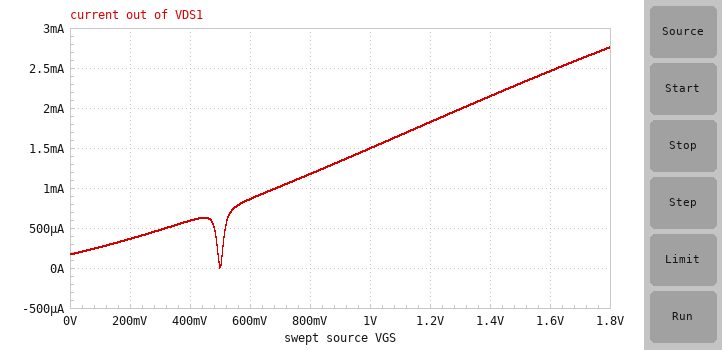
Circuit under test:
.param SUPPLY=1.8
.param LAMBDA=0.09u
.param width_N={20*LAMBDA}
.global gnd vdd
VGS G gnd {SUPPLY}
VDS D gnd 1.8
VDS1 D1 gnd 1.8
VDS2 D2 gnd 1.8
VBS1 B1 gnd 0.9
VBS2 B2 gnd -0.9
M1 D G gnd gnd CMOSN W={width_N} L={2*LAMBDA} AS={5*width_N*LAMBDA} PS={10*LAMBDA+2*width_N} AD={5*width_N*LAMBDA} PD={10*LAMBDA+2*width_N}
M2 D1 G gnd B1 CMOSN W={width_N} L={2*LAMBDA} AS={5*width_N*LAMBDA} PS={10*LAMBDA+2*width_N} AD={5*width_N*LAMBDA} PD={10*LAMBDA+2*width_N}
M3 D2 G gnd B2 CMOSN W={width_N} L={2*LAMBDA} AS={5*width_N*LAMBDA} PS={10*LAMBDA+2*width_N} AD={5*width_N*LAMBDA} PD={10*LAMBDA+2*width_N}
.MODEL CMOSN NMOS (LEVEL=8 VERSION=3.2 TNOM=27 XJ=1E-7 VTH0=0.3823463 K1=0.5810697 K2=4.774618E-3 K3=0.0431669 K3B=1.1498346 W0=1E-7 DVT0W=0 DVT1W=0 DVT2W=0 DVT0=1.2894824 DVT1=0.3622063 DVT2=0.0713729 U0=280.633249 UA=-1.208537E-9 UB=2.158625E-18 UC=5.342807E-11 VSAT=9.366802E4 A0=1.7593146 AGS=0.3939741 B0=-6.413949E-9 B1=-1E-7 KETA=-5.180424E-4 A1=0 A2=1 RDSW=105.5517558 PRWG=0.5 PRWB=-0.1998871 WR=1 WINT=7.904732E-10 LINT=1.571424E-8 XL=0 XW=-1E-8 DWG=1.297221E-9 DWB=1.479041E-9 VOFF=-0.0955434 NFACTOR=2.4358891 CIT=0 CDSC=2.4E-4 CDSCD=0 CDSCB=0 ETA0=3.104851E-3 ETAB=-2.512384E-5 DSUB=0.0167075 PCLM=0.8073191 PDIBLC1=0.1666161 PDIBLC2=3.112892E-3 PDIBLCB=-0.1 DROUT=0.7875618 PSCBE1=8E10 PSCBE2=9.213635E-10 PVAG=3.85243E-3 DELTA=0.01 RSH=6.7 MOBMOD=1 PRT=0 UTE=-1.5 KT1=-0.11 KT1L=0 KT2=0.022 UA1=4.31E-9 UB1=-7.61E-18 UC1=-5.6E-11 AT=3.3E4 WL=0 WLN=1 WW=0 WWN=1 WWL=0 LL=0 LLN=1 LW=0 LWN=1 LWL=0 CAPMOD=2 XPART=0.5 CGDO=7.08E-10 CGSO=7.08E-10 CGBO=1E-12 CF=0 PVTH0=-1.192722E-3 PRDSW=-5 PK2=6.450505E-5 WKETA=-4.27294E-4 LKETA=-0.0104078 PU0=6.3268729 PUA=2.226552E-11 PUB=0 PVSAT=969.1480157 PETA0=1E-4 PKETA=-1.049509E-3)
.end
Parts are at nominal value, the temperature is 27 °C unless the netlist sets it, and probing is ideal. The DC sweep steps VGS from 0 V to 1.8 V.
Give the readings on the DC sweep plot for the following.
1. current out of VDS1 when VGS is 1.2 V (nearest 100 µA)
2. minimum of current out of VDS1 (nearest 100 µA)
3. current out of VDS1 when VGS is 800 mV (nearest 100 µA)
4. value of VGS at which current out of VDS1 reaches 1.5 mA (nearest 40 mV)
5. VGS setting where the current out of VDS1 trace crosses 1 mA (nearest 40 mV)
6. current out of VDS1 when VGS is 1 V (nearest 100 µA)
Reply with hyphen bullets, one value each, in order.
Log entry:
- 1.8 mA
- 0 A
- 1.2 mA
- 1.00 V
- 680 mV
- 1.5 mA
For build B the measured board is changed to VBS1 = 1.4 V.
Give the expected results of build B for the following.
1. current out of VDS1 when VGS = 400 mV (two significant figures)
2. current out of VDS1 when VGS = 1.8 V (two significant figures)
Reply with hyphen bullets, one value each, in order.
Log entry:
- 580 µA
- 2.7 mA
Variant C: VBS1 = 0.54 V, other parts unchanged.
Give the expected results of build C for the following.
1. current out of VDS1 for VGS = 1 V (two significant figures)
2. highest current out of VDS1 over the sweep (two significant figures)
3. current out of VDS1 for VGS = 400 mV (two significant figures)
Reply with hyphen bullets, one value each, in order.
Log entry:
- 1.6 mA
- 2.8 mA
- 610 µA
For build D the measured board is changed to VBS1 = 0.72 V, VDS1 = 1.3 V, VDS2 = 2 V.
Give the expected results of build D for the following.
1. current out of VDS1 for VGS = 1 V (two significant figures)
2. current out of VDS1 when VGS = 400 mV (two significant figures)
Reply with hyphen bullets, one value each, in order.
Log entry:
- 1.2 mA
- 420 µA
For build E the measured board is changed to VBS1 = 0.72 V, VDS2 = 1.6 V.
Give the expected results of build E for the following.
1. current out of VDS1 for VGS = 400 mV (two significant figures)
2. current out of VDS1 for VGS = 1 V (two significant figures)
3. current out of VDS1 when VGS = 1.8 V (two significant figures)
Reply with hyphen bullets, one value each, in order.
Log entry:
- 600 µA
- 1.6 mA
- 2.9 mA
